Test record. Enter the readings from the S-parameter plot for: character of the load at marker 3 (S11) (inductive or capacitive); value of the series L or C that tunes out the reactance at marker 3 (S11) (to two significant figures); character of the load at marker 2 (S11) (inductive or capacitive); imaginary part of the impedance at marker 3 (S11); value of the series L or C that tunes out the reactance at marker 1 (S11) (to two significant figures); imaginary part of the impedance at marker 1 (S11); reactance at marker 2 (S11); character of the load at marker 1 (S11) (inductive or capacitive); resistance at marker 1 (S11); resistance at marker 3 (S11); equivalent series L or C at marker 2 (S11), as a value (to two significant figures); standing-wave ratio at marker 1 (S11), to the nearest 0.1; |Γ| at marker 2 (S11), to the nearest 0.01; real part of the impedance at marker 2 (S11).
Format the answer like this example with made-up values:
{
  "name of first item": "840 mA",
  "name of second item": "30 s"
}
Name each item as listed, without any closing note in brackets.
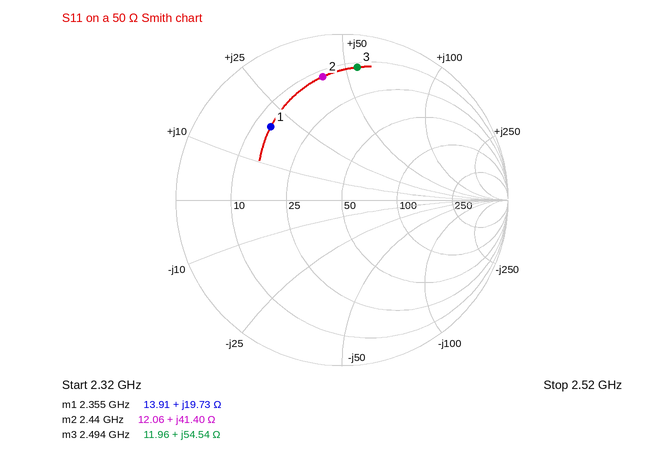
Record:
{
  "character of the load at marker 3 (S11)": "inductive",
  "value of the series L or C that tunes out the reactance at marker 3 (S11)": "1.2 pF",
  "character of the load at marker 2 (S11)": "inductive",
  "imaginary part of the impedance at marker 3": "+54.54 Ω",
  "value of the series L or C that tunes out the reactance at marker 1 (S11)": "3.4 pF",
  "imaginary part of the impedance at marker 1": "+19.73 Ω",
  "reactance at marker 2": "+41.40 Ω",
  "character of the load at marker 1 (S11)": "inductive",
  "resistance at marker 1": "13.91 Ω",
  "resistance at marker 3": "11.96 Ω",
  "equivalent series L or C at marker 2 (S11), as a value": "2.7 nH",
  "standing-wave ratio at marker 1 (S11), to the nearest 0.1": "4.2",
  "|Γ| at marker 2 (S11), to the nearest 0.01": "0.75",
  "real part of the impedance at marker 2": "12.06 Ω"
}
